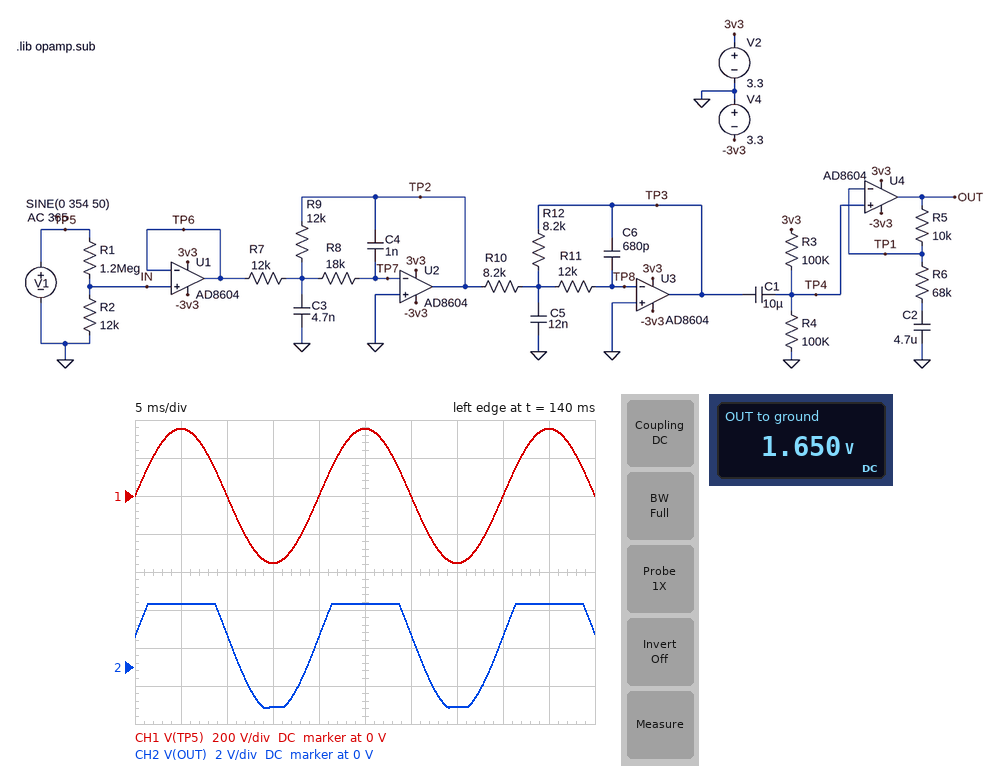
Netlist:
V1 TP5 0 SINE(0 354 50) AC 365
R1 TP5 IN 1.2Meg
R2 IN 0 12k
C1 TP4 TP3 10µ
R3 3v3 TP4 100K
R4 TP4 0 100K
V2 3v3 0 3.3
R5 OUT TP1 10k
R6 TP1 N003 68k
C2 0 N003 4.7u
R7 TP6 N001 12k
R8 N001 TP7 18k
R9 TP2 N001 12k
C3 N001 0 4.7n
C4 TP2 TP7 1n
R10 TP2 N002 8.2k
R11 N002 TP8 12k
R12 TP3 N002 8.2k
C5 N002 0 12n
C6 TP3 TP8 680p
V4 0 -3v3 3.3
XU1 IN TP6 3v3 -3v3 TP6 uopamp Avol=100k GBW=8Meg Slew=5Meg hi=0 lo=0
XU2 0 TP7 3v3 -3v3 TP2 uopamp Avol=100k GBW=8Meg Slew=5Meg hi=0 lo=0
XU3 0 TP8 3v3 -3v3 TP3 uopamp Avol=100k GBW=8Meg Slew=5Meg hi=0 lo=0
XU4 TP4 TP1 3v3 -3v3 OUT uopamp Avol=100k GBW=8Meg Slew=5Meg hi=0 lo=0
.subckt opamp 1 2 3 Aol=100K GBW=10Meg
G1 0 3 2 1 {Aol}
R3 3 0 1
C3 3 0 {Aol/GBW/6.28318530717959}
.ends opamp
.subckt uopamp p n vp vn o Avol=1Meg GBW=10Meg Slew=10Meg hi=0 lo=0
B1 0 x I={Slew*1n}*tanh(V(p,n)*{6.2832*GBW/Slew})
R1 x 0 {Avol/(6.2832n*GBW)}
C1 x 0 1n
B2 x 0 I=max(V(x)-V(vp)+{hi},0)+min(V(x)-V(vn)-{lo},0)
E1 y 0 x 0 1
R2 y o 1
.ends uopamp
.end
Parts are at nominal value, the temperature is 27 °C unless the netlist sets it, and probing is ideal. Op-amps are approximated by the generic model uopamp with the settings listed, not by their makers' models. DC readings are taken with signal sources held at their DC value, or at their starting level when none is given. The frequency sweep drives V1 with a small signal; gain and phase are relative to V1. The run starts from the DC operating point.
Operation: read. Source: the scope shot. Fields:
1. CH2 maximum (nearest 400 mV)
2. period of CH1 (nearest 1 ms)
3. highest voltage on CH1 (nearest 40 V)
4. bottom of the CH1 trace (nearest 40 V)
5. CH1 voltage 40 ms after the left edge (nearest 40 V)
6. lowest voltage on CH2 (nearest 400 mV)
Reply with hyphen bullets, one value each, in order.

- 3.2 V
- 20 ms
- 360 V
- -360 V
- 0 V
- -2.0 V
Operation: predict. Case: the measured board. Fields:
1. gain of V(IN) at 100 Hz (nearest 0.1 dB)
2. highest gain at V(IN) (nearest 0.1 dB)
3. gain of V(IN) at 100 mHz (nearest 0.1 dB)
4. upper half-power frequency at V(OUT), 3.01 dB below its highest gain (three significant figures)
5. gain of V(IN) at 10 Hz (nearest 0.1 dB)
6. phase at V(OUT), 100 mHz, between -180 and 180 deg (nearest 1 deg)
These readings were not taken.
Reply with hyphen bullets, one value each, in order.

- -40.1 dB
- -40.1 dB
- -40.1 dB
- 5.54 kHz
- -40.1 dB
- 74 deg
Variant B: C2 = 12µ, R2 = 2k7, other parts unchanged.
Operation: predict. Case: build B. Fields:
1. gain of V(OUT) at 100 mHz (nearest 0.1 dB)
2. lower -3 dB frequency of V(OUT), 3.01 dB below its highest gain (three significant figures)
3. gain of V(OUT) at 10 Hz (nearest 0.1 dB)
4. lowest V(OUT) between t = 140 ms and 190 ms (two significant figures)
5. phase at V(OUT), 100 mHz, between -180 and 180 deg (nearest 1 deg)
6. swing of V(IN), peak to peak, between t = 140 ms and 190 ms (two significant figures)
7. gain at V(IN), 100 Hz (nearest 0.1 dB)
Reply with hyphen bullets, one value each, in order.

- -63.2 dB
- 415 mHz
- -51.8 dB
- 730 mV
- 76 deg
- 1.6 V
- -53.0 dB
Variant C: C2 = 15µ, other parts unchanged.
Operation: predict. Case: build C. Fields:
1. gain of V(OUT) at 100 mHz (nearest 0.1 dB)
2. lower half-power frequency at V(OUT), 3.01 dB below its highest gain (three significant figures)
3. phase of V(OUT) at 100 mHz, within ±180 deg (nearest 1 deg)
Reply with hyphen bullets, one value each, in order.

- -50.2 dB
- 408 mHz
- 76 deg
